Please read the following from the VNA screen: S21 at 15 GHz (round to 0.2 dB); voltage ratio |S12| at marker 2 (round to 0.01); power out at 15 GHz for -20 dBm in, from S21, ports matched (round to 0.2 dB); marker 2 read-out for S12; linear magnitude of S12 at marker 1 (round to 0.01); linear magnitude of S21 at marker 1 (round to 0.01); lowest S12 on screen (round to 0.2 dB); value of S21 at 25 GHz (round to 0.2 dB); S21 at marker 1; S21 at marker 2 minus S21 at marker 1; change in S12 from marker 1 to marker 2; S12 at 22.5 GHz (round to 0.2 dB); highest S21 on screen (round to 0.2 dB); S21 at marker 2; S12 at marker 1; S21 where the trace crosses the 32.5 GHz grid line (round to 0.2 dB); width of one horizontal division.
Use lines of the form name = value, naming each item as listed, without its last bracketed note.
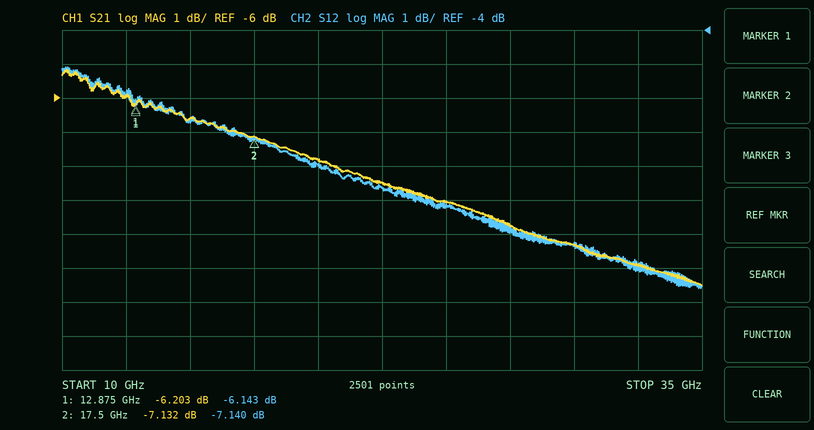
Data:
S21 at 15 GHz = -6.6 dB
voltage ratio |S12| at marker 2 = 0.44
power out at 15 GHz for -20 dBm in, from S21, ports matched = -26.6 dBm
marker 2 read-out for S12 = -7.140 dB
linear magnitude of S12 at marker 1 = 0.49
linear magnitude of S21 at marker 1 = 0.49
lowest S12 on screen = -11.6 dB
value of S21 at 25 GHz = -9.0 dB
S21 at marker 1 = -6.203 dB
S21 at marker 2 minus S21 at marker 1 = -0.929 dB
change in S12 from marker 1 to marker 2 = -0.997 dB
S12 at 22.5 GHz = -8.6 dB
highest S21 on screen = -5.2 dB
S21 at marker 2 = -7.132 dB
S12 at marker 1 = -6.143 dB
S21 where the trace crosses the 32.5 GHz grid line = -11.0 dB
width of one horizontal division = 2.5 GHz
